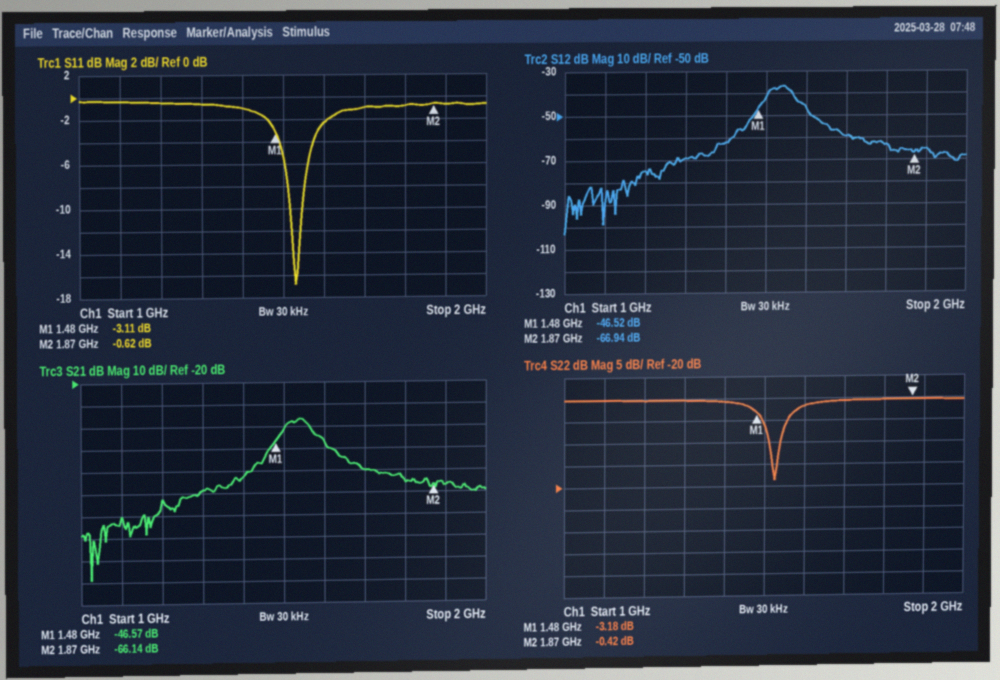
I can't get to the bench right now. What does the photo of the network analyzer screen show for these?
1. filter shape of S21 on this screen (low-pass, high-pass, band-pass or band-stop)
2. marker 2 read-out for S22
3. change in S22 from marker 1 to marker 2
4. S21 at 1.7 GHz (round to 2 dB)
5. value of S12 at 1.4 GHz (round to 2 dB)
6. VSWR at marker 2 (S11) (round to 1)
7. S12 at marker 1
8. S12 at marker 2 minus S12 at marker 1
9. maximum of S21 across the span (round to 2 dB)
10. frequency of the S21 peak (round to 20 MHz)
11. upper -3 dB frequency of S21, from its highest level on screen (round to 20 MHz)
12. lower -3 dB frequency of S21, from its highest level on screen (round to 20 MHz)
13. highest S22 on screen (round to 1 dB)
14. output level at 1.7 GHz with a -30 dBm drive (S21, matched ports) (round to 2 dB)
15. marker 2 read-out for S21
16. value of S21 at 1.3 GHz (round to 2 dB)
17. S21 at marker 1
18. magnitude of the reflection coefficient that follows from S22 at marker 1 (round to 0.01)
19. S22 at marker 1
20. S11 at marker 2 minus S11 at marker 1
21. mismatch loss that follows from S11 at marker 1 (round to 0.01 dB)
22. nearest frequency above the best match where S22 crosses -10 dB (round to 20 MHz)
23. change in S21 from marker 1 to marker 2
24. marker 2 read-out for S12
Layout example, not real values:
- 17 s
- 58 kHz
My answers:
- band-pass
- -0.42 dB
- 2.76 dB
- -60 dB
- -62 dB
- 28
- -46.52 dB
- -20.42 dB
- -36 dB
- 1.54 GHz
- 1.56 GHz
- 1.50 GHz
- 0 dB
- -90 dBm
- -66.14 dB
- -68 dB
- -46.57 dB
- 0.69
- -3.18 dB
- 2.49 dB
- 2.91 dB
- 1.54 GHz
- -19.57 dB
- -66.94 dB
